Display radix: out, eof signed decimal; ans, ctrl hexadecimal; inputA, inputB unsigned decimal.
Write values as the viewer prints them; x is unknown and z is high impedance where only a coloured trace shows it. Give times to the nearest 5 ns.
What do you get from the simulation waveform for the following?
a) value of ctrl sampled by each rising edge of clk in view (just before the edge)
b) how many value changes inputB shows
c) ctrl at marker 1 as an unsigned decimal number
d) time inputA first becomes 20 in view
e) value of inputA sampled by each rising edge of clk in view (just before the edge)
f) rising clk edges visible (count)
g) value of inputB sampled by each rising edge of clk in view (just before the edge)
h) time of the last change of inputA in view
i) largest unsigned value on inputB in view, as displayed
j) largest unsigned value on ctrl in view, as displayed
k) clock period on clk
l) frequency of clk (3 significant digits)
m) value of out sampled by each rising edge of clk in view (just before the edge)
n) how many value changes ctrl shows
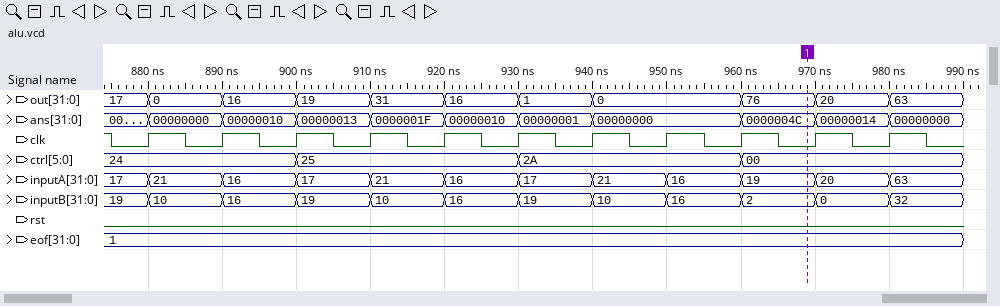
24, 24, 24, 25, 25, 25, 2A, 2A, 2A, 00, 00
11
0
970 ns
17, 21, 16, 17, 21, 16, 17, 21, 16, 19, 20
11
19, 10, 16, 19, 10, 16, 19, 10, 16, 2, 0
980 ns
32
2A
10 ns
100 MHz
17, 0, 16, 19, 31, 16, 1, 0, 0, 76, 20
3
